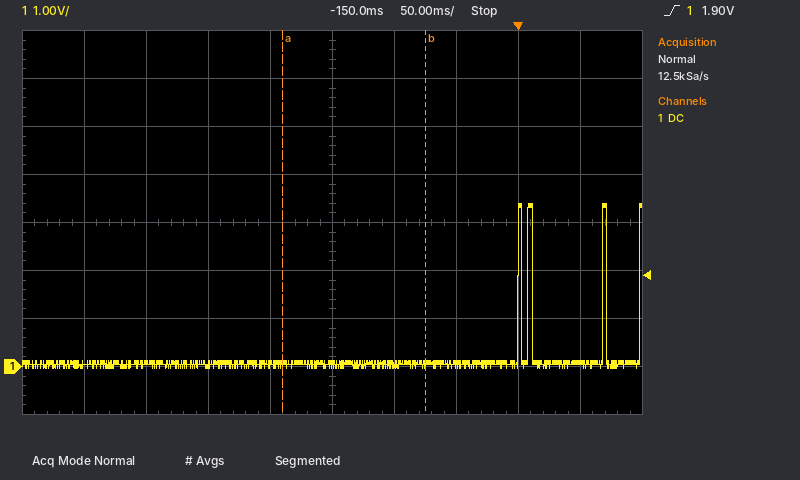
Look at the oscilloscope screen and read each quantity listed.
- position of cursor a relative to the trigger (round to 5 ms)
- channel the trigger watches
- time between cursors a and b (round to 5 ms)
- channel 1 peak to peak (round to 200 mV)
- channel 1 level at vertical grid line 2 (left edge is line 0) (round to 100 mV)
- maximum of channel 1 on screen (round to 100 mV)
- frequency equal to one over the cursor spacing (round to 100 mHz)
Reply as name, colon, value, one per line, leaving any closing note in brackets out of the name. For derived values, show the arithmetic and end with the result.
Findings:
position of cursor a relative to the trigger: -190 ms
channel the trigger watches: channel 1
time between cursors a and b: 115 ms
channel 1 peak to peak: 3.4 V
channel 1 level at vertical grid line 2 (left edge is line 0): 100 mV
maximum of channel 1 on screen: 3.4 V
frequency equal to one over the cursor spacing: 1 / 115 ms ≈ 8.7 Hz
